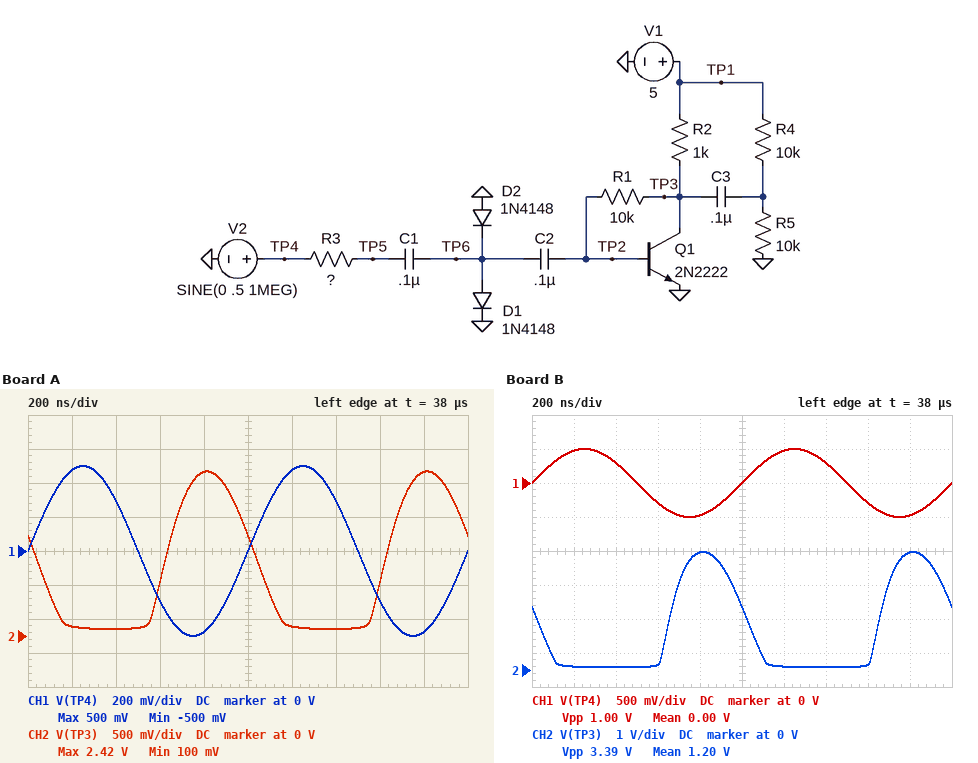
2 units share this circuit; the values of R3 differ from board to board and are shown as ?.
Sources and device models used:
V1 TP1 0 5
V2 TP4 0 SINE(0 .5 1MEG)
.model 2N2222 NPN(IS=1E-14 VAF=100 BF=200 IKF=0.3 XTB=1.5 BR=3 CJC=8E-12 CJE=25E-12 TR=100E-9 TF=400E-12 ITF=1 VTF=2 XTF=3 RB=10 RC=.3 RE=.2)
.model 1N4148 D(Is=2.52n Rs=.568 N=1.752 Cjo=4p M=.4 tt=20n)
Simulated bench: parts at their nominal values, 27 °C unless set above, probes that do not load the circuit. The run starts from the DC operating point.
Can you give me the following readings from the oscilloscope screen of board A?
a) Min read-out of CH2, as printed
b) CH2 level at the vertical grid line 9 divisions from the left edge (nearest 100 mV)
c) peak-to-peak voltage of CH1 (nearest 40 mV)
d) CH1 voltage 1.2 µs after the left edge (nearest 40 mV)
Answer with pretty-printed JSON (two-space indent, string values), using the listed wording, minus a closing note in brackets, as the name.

{
  "Min read-out of CH2, as printed": "100 mV",
  "CH2 level at the vertical grid line 9 divisions from the left edge": "2.4 V",
  "peak-to-peak voltage of CH1": "1.00 V",
  "CH1 voltage 1.2 µs after the left edge": "480 mV"
}
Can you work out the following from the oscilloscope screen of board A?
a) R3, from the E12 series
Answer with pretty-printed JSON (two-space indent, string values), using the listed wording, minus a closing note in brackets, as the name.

{
  "R3, from the E12 series": "2.7 kΩ"
}
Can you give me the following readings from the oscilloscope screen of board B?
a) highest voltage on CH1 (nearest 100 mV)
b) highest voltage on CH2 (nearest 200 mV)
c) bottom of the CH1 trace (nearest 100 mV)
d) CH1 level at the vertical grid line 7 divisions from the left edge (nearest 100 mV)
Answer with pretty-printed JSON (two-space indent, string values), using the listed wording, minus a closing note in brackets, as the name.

{
  "highest voltage on CH1": "500 mV",
  "highest voltage on CH2": "3.4 V",
  "bottom of the CH1 trace": "-500 mV",
  "CH1 level at the vertical grid line 7 divisions from the left edge": "300 mV"
}
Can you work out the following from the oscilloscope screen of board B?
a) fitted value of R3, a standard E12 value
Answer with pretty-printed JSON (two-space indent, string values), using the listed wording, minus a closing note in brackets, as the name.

{
  "fitted value of R3, a standard E12 value": "1.5 kΩ"
}
